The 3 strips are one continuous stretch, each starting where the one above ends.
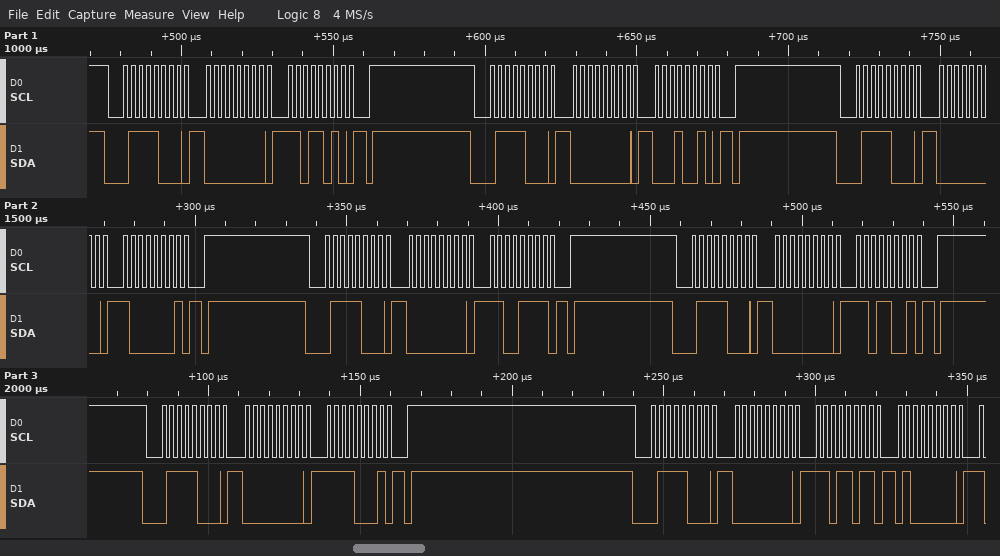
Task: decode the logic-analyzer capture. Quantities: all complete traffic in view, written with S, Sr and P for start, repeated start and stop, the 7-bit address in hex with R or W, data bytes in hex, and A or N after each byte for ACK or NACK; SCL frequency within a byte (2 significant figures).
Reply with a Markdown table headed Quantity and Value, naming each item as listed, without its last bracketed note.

| Quantity | Value |
|---|---|
| all complete traffic in view, written with S, Sr and P for start, repeated start and stop, the 7-bit address in hex with R or W, data bytes in hex, and A or N after each byte for ACK or NACK | S 3CW A 00 A DA A P S 3CW A 00 A 12 A P S 3CW A 00 A 81 A P S 3CW A 00 A CF A P S 3CW A 00 A D9 A P S 3CW A 00 A F1 A P S 3CW A 00 A DB A 40 A |
| SCL frequency within a byte | 400 kHz |
